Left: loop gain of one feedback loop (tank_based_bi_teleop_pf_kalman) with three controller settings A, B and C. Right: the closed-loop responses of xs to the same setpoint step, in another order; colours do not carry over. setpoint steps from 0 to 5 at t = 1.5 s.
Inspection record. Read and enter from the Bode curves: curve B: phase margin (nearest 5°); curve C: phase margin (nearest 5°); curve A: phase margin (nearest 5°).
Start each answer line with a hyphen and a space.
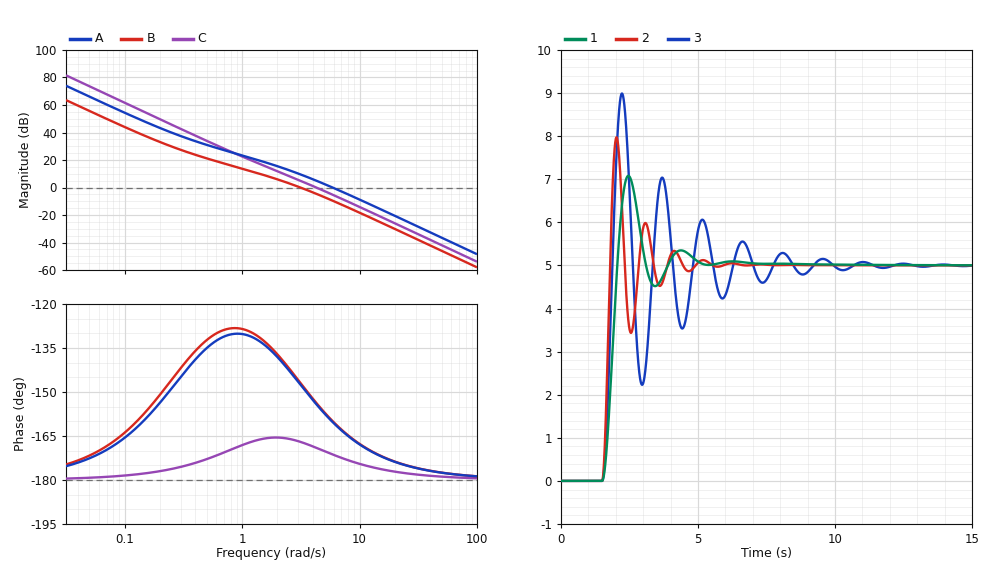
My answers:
- 35°
- 10°
- 20°
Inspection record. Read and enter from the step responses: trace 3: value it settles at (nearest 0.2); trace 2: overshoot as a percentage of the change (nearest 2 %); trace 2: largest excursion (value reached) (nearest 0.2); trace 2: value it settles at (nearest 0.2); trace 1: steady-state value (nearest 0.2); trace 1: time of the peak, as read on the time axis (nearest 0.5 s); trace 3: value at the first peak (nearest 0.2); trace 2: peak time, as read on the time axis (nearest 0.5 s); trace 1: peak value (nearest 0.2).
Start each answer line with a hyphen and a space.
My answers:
- 5.0
- 60 %
- 8.0
- 5.0
- 5.0
- 2.5 s
- 9.0
- 2.0 s
- 7.0
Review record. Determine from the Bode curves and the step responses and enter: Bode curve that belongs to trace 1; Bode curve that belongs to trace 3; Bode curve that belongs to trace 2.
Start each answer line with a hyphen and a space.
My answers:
- B
- C
- A
